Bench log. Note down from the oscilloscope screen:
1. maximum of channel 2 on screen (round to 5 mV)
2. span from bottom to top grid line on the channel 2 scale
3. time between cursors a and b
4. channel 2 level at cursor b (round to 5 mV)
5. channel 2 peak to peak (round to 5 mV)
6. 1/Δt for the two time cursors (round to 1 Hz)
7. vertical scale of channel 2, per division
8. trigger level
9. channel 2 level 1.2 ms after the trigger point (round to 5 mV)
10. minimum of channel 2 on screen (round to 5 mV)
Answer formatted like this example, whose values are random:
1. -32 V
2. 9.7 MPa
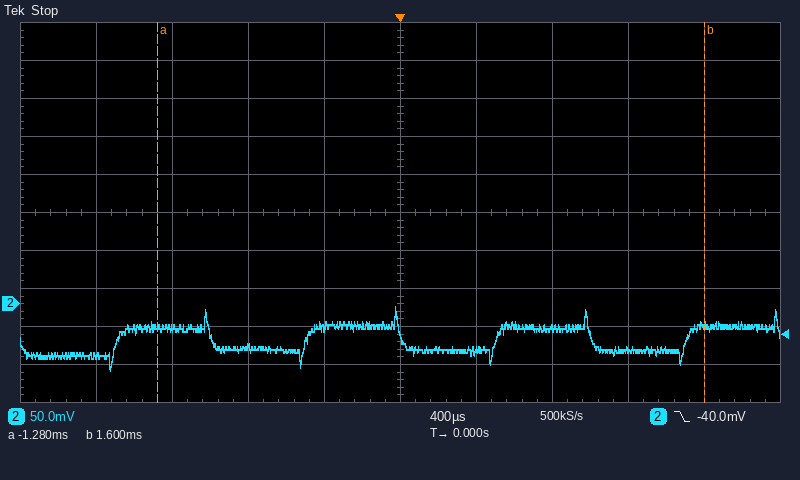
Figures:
1. -5 mV
2. 500 mV
3. 2.88 ms
4. -30 mV
5. 85 mV
6. 347 Hz
7. 50 mV
8. -40.0 mV
9. -60 mV
10. -90 mV
